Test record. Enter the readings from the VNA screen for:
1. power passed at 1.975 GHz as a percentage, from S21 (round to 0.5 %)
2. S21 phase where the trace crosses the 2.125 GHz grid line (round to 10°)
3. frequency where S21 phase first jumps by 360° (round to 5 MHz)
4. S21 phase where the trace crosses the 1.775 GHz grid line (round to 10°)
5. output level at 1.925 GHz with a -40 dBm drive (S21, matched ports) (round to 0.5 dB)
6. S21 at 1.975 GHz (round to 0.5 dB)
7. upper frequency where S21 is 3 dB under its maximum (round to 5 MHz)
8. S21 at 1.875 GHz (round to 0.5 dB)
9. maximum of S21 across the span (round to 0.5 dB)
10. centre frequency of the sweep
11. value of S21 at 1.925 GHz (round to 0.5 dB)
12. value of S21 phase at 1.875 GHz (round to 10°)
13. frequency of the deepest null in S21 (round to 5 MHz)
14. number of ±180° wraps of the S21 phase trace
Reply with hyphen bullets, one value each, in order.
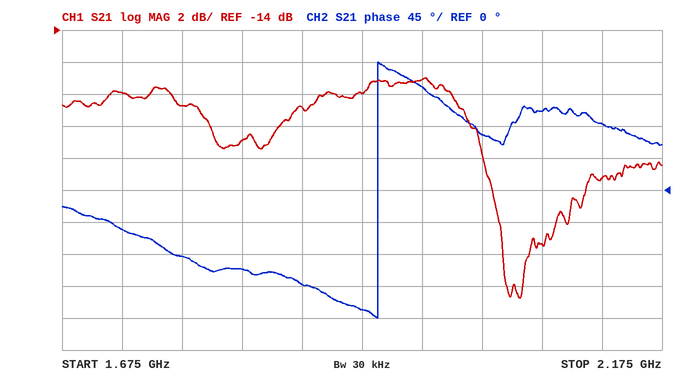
- 2.0 %
- 90°
- 1.940 GHz
- -90°
- -58.0 dBm
- -17.0 dB
- 2.015 GHz
- -19.0 dB
- -17.0 dB
- 1.925 GHz
- -18.0 dB
- -130°
- 2.055 GHz
- 1
